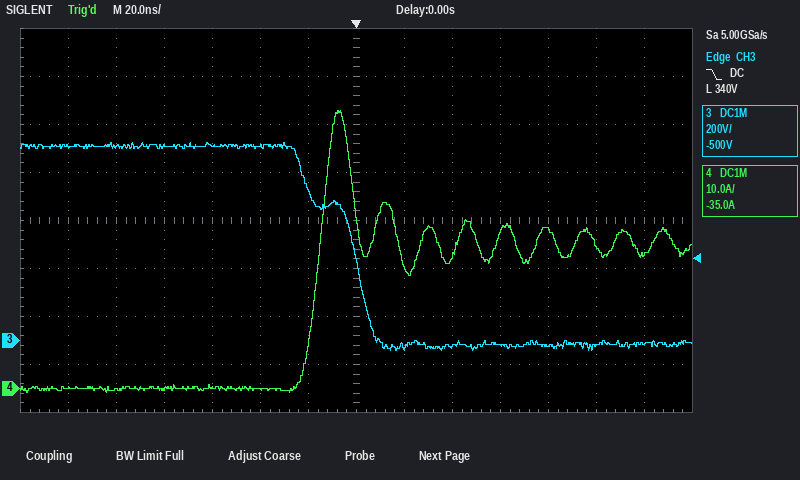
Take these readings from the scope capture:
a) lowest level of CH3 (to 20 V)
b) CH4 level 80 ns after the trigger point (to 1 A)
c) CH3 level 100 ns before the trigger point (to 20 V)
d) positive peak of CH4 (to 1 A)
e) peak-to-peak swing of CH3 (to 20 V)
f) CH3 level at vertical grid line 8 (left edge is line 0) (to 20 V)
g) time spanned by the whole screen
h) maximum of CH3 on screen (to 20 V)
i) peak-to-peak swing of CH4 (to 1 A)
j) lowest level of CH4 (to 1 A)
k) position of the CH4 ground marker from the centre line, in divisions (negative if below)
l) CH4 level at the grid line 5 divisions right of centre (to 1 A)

-40 V
33 A
800 V
58 A
860 V
-20 V
280 ns
820 V
59 A
-1 A
-3.5 div
30 A
